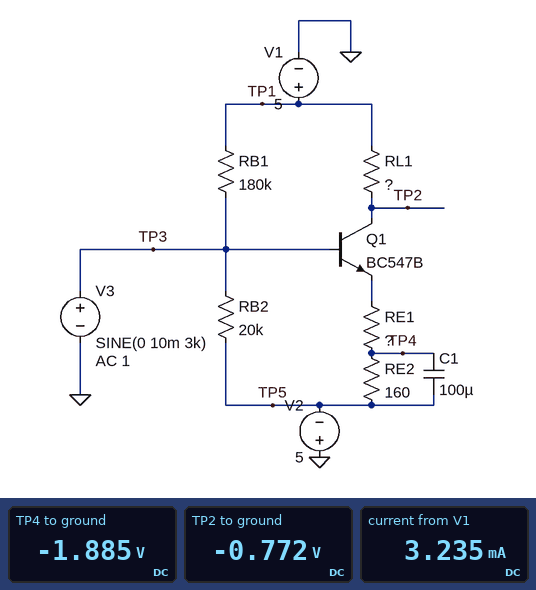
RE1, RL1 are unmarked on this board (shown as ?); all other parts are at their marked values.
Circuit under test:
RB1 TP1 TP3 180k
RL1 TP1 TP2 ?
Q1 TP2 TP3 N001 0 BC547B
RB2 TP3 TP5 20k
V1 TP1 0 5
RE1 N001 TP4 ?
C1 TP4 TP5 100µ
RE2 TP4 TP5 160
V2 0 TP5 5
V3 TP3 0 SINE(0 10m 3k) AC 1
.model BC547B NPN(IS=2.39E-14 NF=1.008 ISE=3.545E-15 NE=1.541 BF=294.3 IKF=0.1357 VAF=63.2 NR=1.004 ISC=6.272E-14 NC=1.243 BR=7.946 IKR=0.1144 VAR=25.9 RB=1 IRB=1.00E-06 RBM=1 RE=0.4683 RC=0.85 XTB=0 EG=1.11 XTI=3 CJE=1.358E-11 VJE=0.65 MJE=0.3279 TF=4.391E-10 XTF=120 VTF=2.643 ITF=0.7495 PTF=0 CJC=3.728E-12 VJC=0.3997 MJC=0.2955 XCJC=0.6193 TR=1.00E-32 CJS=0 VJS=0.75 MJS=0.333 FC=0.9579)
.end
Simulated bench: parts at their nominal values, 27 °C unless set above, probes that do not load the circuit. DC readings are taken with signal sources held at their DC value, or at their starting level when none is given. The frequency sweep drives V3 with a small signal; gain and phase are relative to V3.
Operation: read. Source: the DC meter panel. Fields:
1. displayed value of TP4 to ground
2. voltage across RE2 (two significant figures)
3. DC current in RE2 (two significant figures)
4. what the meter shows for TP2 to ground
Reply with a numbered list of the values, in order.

1. -1.885 V
2. 3.1 V
3. 19 mA
4. -0.772 V
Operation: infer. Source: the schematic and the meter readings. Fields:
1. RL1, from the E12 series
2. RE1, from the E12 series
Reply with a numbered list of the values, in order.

1. 1.8 kΩ
2. 56 Ω
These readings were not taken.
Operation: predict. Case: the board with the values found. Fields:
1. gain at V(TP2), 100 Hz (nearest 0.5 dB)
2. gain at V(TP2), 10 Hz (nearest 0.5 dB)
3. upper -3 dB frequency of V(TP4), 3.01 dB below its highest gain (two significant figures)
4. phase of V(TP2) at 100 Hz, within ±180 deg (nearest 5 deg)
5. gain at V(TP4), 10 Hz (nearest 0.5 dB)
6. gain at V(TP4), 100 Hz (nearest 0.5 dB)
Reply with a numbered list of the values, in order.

1. -0.5 dB
2. 0 dB
3. 37 Hz
4. 0 deg
5. -3.0 dB
6. -12.0 dB
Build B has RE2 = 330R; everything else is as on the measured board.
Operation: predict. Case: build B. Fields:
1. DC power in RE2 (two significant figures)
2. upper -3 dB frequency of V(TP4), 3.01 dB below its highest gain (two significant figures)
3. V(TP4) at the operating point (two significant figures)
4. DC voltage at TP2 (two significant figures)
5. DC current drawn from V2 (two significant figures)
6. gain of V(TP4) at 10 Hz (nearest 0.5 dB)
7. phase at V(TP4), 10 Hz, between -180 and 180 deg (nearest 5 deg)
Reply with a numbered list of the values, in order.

1. 40 mW
2. 31 Hz
3. -1.4 V
4. -740 mV
5. 11 mA
6. -2.0 dB
7. -20 deg
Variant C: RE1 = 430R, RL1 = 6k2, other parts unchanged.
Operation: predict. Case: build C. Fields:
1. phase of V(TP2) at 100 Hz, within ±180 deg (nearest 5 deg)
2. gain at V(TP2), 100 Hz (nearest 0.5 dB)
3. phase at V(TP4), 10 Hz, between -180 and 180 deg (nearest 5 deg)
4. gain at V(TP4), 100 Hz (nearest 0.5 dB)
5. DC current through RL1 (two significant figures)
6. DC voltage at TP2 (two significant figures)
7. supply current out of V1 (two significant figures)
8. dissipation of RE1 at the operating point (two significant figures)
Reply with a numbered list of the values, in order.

1. 0 deg
2. 0 dB
3. -35 deg
4. -29.0 dB
5. 930 µA
6. -740 mV
7. 950 µA
8. 22 mW
